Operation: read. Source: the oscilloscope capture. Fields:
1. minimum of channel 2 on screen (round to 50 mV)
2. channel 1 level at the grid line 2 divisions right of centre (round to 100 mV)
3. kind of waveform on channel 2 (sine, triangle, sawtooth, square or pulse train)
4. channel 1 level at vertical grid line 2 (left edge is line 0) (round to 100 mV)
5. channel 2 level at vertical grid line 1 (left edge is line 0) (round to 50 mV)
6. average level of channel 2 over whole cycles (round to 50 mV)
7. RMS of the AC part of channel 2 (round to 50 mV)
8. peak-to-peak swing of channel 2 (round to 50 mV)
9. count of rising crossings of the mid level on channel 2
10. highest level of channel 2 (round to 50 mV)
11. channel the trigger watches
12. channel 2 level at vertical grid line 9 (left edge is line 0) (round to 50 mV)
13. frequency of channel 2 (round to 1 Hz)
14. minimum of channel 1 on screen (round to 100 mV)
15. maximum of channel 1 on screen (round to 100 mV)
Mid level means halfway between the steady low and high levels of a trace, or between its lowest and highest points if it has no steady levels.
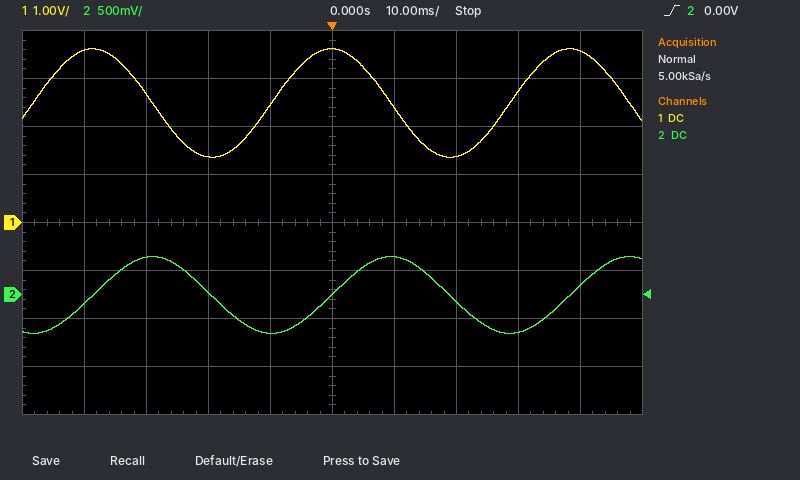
-400 mV
1.4 V
sine
2.7 V
-100 mV
0 mV
300 mV
800 mV
3
400 mV
channel 2
100 mV
26 Hz
1.4 V
3.6 V
